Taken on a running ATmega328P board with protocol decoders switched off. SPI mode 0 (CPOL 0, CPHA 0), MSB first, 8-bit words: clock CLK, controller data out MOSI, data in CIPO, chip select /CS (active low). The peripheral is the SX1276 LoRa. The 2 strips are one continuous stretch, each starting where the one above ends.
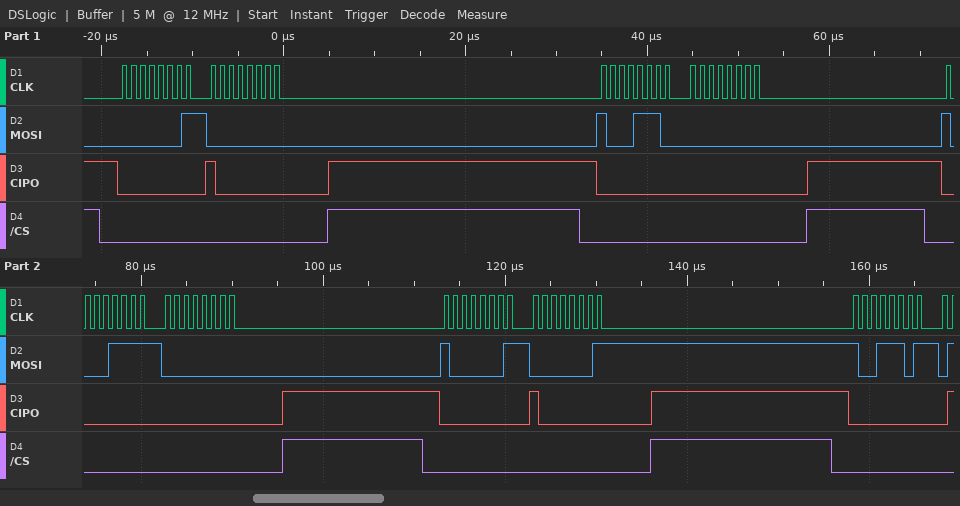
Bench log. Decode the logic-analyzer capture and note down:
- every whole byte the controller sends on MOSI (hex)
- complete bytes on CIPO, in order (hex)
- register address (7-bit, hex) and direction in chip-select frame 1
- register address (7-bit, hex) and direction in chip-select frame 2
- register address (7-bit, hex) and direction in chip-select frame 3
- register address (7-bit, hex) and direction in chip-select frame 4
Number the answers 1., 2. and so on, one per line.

1. 01 00 8E 00 8F 00 81 01 9D
2. 00 80 00 00 00 00 00 80 00
3. 0x01 read
4. 0x0E write
5. 0x0F write
6. 0x01 write
